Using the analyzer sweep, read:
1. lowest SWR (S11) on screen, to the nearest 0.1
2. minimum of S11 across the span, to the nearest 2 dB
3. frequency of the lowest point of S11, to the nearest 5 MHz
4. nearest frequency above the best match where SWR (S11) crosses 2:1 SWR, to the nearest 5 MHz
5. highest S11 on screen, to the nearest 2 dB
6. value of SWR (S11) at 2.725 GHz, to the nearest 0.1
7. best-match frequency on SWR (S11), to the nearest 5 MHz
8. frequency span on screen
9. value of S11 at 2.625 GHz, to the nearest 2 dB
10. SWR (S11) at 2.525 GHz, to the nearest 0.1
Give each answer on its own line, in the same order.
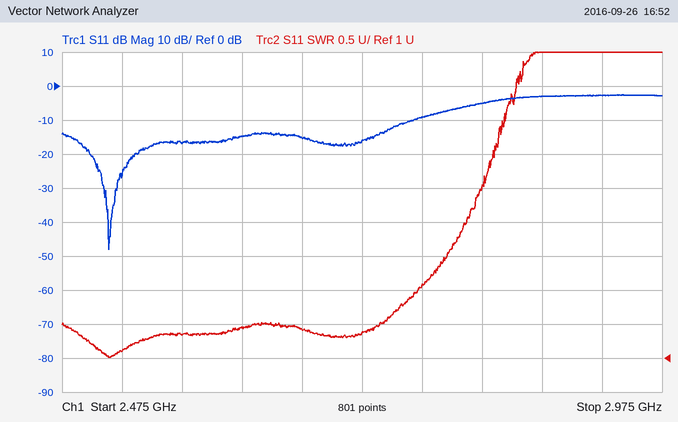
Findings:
1.0
-48 dB
2.515 GHz
2.770 GHz
-2 dB
1.4
2.515 GHz
500 MHz
-14 dB
1.1
